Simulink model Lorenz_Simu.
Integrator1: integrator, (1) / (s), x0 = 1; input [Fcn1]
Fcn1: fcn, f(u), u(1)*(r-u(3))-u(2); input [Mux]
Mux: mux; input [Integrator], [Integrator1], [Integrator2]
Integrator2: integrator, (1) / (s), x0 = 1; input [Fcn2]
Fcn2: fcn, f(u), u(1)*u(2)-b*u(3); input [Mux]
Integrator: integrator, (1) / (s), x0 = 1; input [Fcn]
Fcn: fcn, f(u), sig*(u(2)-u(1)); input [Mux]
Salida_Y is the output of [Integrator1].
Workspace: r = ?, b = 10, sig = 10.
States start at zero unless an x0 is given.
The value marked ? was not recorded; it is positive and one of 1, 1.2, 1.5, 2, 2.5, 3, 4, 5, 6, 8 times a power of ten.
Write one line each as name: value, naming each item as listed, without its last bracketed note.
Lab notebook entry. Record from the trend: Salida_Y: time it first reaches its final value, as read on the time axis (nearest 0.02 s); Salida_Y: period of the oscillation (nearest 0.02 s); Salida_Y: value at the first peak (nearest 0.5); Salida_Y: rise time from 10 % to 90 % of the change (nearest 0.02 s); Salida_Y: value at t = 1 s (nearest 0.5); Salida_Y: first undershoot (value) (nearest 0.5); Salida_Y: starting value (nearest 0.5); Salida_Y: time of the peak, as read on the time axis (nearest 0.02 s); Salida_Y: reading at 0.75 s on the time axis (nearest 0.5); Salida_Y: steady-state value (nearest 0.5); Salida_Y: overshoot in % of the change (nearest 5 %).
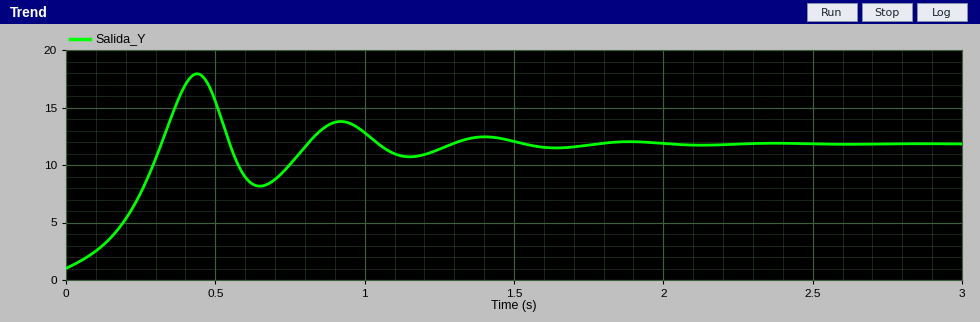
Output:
Salida_Y: time it first reaches its final value, as read on the time axis: 0.32 s
Salida_Y: period of the oscillation: 0.48 s
Salida_Y: value at the first peak: 18.0
Salida_Y: rise time from 10 % to 90 % of the change: 0.22 s
Salida_Y: value at t = 1 s: 13.0
Salida_Y: first undershoot (value): 8.0
Salida_Y: starting value: 1.0
Salida_Y: time of the peak, as read on the time axis: 0.44 s
Salida_Y: reading at 0.75 s on the time axis: 10.0
Salida_Y: steady-state value: 12.0
Salida_Y: overshoot in % of the change: 55 %
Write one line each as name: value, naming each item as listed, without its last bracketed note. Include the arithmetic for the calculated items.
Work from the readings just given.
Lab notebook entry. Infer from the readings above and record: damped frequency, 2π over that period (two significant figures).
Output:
damped frequency, 2π over that period: 2π / 0.48 = 13 rad/s
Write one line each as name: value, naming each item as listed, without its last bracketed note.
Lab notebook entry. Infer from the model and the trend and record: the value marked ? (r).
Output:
the value marked ?: 15
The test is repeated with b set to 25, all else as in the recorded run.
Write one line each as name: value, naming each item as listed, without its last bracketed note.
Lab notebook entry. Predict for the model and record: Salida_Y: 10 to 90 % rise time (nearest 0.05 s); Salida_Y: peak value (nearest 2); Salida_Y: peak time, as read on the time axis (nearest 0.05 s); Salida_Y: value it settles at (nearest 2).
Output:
Salida_Y: 10 to 90 % rise time: 0.25 s
Salida_Y: peak value: 24
Salida_Y: peak time, as read on the time axis: 0.50 s
Salida_Y: value it settles at: 18
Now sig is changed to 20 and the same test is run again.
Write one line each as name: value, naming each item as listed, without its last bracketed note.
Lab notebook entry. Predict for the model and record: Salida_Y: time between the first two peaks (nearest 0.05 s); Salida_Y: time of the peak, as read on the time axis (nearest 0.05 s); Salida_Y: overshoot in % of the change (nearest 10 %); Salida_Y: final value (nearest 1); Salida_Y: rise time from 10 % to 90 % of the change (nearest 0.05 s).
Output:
Salida_Y: time between the first two peaks: 0.45 s
Salida_Y: time of the peak, as read on the time axis: 0.35 s
Salida_Y: overshoot in % of the change: 50 %
Salida_Y: final value: 12
Salida_Y: rise time from 10 % to 90 % of the change: 0.20 s
